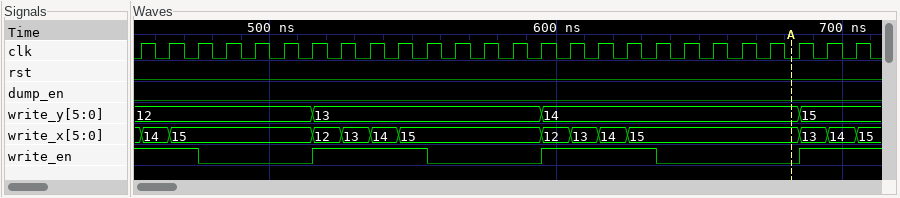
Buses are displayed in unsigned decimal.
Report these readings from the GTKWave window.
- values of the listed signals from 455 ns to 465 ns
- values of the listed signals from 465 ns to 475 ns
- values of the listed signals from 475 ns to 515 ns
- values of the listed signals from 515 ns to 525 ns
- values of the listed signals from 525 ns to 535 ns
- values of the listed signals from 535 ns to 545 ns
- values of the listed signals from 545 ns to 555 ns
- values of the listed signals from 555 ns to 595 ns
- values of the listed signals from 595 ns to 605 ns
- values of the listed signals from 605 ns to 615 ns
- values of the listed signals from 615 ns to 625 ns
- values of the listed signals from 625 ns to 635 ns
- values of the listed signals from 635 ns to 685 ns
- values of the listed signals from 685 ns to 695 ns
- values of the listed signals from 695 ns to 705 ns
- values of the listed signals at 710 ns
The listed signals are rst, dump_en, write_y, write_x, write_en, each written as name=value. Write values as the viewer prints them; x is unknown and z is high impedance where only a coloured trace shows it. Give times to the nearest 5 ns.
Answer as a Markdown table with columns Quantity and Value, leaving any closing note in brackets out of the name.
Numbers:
| Quantity | Value |
|---|---|
| values of the listed signals from 455 ns to 465 ns | rst=0, dump_en=0, write_y=12, write_x=14, write_en=1 |
| values of the listed signals from 465 ns to 475 ns | rst=0, dump_en=0, write_y=12, write_x=15, write_en=1 |
| values of the listed signals from 475 ns to 515 ns | rst=0, dump_en=0, write_y=12, write_x=15, write_en=0 |
| values of the listed signals from 515 ns to 525 ns | rst=0, dump_en=0, write_y=13, write_x=12, write_en=1 |
| values of the listed signals from 525 ns to 535 ns | rst=0, dump_en=0, write_y=13, write_x=13, write_en=1 |
| values of the listed signals from 535 ns to 545 ns | rst=0, dump_en=0, write_y=13, write_x=14, write_en=1 |
| values of the listed signals from 545 ns to 555 ns | rst=0, dump_en=0, write_y=13, write_x=15, write_en=1 |
| values of the listed signals from 555 ns to 595 ns | rst=0, dump_en=0, write_y=13, write_x=15, write_en=0 |
| values of the listed signals from 595 ns to 605 ns | rst=0, dump_en=0, write_y=14, write_x=12, write_en=1 |
| values of the listed signals from 605 ns to 615 ns | rst=0, dump_en=0, write_y=14, write_x=13, write_en=1 |
| values of the listed signals from 615 ns to 625 ns | rst=0, dump_en=0, write_y=14, write_x=14, write_en=1 |
| values of the listed signals from 625 ns to 635 ns | rst=0, dump_en=0, write_y=14, write_x=15, write_en=1 |
| values of the listed signals from 635 ns to 685 ns | rst=0, dump_en=0, write_y=14, write_x=15, write_en=0 |
| values of the listed signals from 685 ns to 695 ns | rst=0, dump_en=0, write_y=15, write_x=13, write_en=1 |
| values of the listed signals from 695 ns to 705 ns | rst=0, dump_en=0, write_y=15, write_x=14, write_en=1 |
| values of the listed signals at 710 ns | rst=0, dump_en=0, write_y=15, write_x=15, write_en=1 |
